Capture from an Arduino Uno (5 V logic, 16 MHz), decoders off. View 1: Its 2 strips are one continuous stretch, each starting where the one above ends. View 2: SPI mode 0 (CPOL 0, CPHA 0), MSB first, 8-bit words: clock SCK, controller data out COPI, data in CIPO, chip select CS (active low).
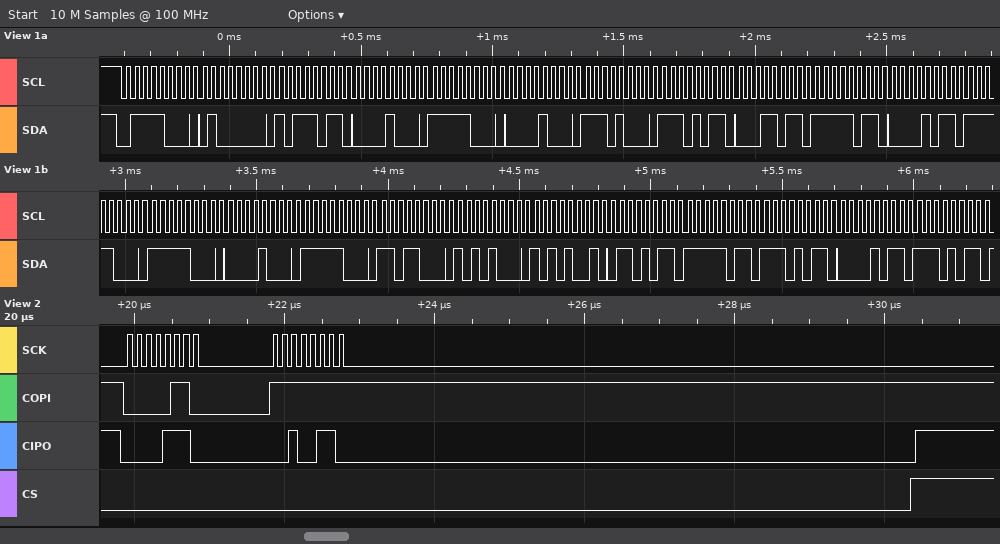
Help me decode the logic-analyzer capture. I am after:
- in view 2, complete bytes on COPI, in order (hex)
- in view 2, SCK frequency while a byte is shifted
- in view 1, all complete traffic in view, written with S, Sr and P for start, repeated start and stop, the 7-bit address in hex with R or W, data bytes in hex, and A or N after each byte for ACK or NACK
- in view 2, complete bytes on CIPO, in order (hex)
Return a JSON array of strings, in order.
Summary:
["06 FF", "8 MHz", "S 3CW A 40 A BB A 08 A F8 A 08 A E8 A EB A 1B A FB A 0B A F8 A F8 A 08 A F8 A D8 A A8 A A9 A 6B A FB A EB A 0B A EB A", "0E 26"]
